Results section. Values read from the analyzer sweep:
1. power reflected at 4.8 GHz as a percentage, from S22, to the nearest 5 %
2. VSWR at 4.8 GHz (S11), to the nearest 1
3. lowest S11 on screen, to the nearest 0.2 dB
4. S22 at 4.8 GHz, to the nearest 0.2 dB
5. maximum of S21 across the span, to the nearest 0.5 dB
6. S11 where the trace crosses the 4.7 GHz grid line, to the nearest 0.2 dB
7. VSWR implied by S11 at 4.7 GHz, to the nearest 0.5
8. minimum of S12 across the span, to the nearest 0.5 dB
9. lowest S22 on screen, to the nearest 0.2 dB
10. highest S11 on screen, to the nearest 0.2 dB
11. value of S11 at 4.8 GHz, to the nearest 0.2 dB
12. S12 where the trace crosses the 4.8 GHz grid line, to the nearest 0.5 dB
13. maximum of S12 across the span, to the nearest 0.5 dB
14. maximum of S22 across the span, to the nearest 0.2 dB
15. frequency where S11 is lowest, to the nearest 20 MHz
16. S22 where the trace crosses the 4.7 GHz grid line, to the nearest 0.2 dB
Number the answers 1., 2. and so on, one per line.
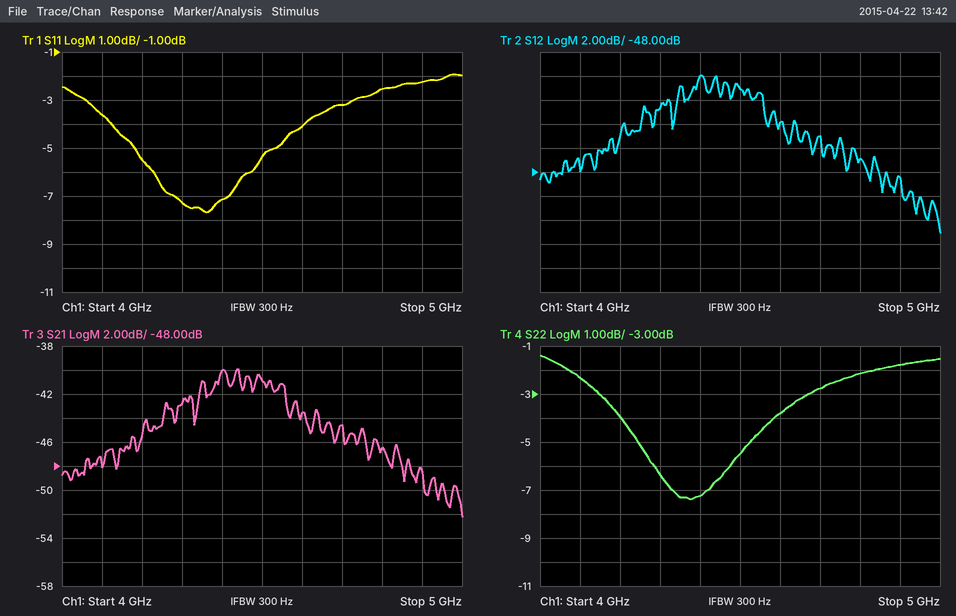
1. 60 %
2. 7
3. -7.6 dB
4. -2.2 dB
5. -40.0 dB
6. -3.2 dB
7. 5.5
8. -53.0 dB
9. -7.4 dB
10. -2.0 dB
11. -2.6 dB
12. -47.0 dB
13. -40.0 dB
14. -1.4 dB
15. 4.36 GHz
16. -2.8 dB
